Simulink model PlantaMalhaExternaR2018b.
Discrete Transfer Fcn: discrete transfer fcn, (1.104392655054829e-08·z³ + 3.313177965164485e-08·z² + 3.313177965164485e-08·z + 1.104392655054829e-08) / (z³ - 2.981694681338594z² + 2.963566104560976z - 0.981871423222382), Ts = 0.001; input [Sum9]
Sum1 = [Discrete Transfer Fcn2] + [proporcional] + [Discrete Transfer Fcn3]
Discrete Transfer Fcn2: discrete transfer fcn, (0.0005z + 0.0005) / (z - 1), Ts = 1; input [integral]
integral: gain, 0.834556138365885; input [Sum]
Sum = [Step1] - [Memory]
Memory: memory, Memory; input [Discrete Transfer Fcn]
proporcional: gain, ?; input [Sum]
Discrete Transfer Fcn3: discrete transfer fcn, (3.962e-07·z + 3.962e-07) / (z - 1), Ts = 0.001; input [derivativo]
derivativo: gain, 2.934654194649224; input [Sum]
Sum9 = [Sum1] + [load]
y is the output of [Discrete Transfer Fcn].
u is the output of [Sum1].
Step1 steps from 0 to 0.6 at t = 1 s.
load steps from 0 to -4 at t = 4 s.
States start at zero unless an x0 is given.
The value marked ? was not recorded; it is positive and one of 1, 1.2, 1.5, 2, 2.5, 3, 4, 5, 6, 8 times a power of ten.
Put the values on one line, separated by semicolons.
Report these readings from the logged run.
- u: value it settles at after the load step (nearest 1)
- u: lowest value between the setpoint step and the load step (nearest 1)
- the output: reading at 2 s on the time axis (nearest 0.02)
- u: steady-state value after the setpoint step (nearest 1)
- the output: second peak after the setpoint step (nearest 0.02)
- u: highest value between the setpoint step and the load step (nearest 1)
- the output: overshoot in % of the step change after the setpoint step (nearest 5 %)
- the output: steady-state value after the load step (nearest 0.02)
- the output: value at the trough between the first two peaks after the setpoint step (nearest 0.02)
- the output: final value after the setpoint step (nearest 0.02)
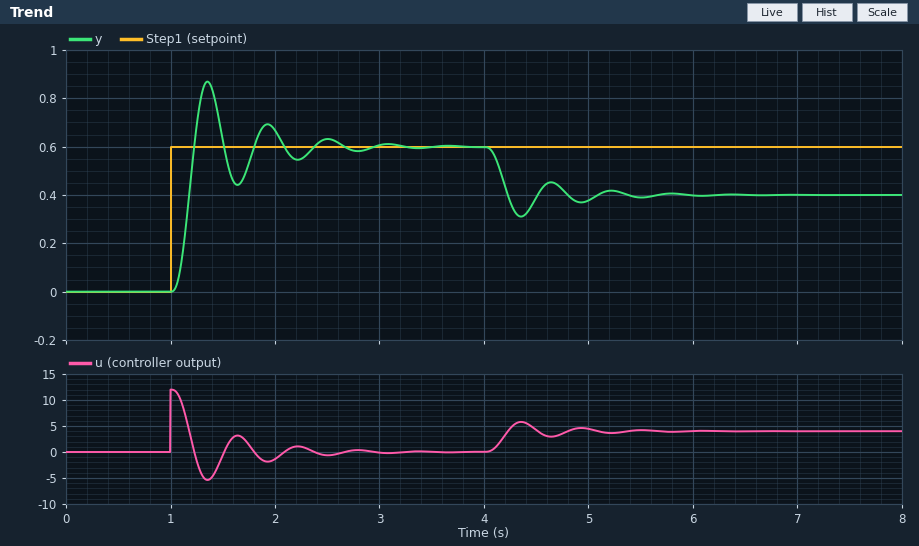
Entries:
4; -5; 0.66; 0; 0.70; 12; 45 %; 0.40; 0.44; 0.60
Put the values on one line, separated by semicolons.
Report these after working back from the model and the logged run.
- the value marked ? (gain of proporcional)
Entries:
20
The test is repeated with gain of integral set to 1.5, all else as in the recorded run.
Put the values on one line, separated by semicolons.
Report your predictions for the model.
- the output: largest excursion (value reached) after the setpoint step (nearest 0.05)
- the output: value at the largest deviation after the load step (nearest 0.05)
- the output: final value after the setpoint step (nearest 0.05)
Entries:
0.85; 0.30; 0.60
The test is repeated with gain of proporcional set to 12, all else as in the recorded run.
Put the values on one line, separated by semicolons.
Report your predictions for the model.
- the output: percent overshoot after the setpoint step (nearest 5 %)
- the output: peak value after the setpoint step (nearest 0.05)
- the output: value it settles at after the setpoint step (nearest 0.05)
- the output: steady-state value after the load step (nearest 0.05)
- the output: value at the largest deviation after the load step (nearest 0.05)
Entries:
20 %; 0.70; 0.60; 0.25; 0.20
